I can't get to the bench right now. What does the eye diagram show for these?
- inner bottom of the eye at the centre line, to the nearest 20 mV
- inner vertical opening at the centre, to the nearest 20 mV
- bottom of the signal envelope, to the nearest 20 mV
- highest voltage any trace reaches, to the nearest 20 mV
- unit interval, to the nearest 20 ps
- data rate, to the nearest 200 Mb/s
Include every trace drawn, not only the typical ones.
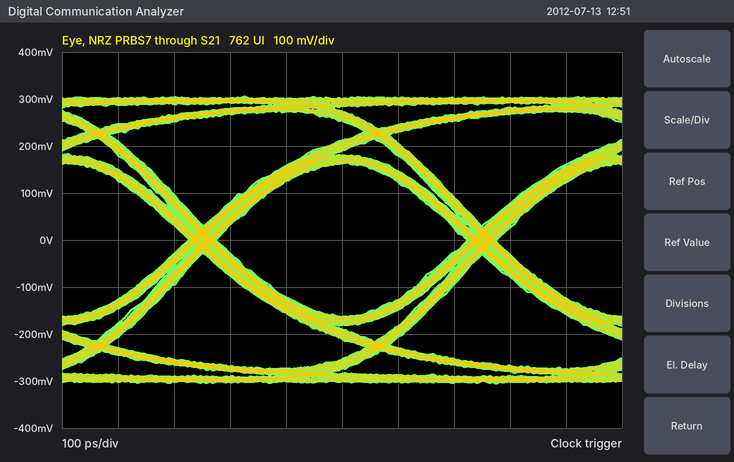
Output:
-160 mV
320 mV
-300 mV
300 mV
500 ps
2.0 Gb/s
